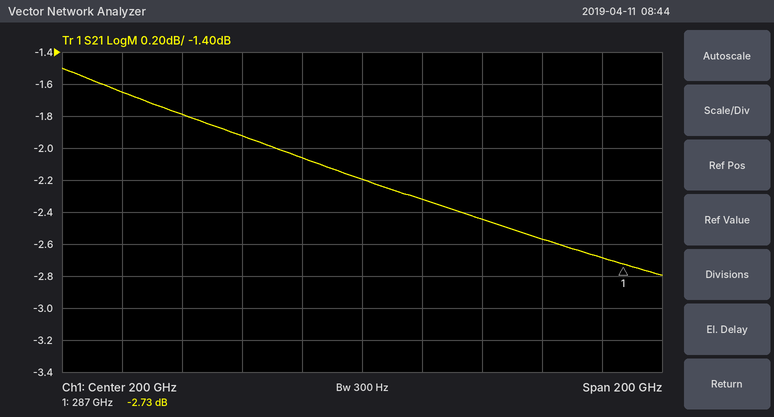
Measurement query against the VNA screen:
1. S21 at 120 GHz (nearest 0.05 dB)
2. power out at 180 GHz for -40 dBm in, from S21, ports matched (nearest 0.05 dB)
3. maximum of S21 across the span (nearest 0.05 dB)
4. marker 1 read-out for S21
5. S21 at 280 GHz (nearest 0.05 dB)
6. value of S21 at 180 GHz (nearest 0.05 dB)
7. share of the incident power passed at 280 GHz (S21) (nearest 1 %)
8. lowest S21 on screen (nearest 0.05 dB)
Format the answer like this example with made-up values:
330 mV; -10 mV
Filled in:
-1.65 dB; -42.05 dBm; -1.50 dB; -2.73 dB; -2.70 dB; -2.05 dB; 54 %; -2.80 dB
